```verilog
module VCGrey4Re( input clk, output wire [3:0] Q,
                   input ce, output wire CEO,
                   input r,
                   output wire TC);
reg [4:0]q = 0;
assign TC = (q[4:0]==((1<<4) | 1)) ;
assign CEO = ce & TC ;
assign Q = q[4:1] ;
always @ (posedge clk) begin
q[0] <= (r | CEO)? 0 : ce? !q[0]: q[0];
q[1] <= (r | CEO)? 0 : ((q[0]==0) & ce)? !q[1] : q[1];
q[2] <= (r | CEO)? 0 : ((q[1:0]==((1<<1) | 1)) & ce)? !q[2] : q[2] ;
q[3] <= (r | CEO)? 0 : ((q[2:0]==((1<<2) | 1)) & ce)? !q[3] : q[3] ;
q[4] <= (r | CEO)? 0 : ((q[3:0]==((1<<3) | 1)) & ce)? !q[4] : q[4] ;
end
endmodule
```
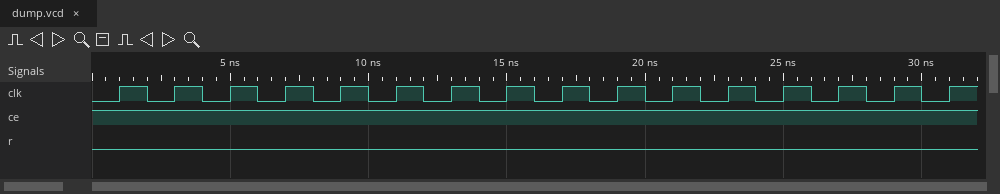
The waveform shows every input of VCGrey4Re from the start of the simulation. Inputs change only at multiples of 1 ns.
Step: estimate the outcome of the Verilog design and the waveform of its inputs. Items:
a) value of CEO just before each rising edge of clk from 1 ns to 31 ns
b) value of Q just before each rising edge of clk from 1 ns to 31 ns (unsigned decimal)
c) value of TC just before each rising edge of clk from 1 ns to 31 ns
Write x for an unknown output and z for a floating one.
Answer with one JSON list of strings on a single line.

["0 0 0 0 0 0 0 0 0 0 0 0 0 0 0 1", "0, 1, 3, 2, 6, 7, 5, 4, 12, 13, 15, 14, 10, 11, 9, 8", "0 0 0 0 0 0 0 0 0 0 0 0 0 0 0 1"]
